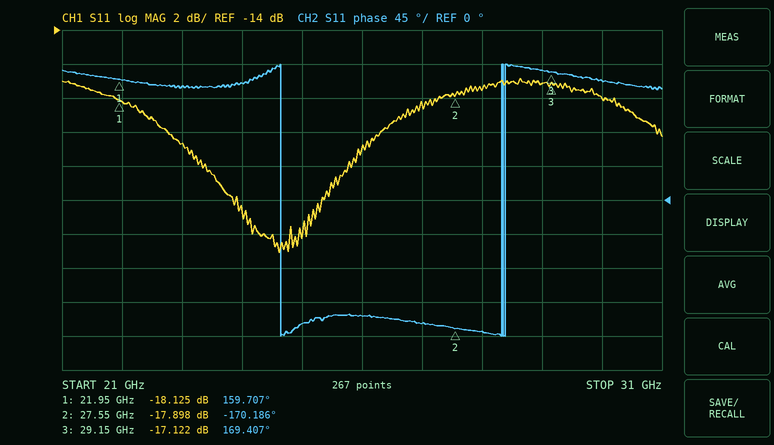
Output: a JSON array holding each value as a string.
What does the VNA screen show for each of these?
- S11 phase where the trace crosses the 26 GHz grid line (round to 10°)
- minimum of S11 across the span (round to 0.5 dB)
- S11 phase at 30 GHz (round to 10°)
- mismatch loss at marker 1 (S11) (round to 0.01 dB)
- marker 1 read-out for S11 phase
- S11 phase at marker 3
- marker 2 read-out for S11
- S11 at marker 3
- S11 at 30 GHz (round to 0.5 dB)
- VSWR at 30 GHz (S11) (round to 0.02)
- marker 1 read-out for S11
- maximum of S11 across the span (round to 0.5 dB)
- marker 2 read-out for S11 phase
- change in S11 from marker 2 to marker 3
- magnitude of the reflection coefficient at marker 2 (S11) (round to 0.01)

["-150°", "-27.0 dB", "160°", "0.07 dB", "159.707°", "169.407°", "-17.898 dB", "-17.122 dB", "-18.0 dB", "1.28", "-18.125 dB", "-17.0 dB", "-170.186°", "0.776 dB", "0.13"]
